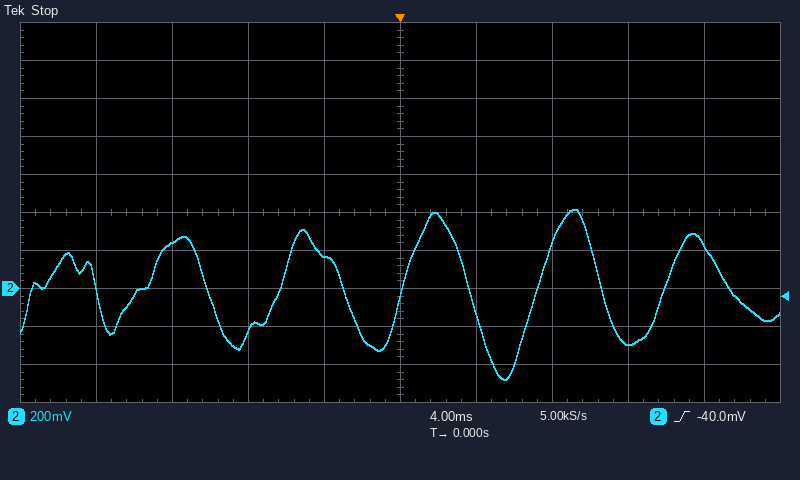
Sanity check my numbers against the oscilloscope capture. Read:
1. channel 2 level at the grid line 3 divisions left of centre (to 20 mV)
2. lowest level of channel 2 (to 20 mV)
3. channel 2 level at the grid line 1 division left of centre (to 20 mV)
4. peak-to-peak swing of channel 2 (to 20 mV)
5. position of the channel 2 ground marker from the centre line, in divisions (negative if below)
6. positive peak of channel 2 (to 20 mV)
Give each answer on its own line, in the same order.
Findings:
240 mV
-480 mV
180 mV
900 mV
-2.0 div
420 mV
